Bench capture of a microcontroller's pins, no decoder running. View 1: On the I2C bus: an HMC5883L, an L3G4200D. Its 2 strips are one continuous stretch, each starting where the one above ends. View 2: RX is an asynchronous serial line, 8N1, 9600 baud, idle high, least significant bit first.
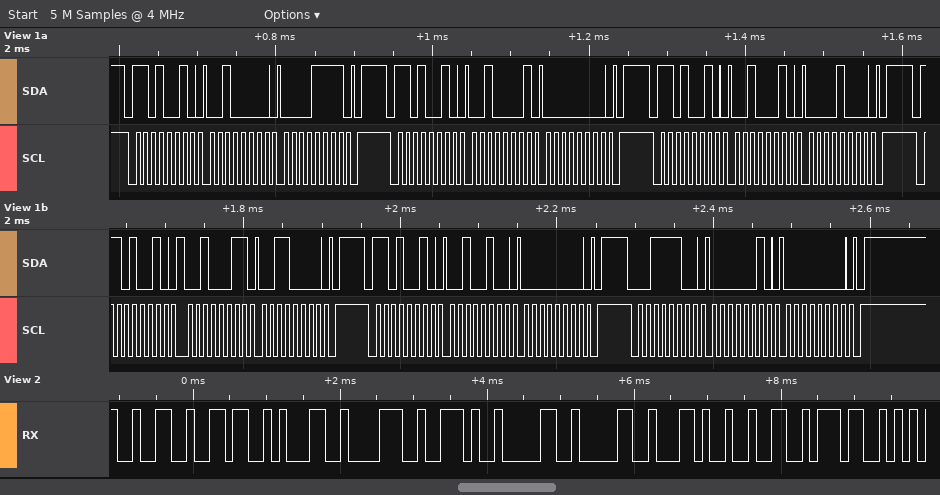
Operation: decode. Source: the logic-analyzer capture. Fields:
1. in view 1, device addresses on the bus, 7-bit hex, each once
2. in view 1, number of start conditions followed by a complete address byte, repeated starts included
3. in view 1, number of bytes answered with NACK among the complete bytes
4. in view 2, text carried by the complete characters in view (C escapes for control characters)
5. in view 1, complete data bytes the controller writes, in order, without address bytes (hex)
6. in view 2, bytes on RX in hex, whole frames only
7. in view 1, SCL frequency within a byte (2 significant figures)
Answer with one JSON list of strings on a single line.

["0x69 0x1E", "6", "0", "\"2618.00,27\"", "20 0F 21 00 22 08 23 30 24 00 02 00", "32 36 31 38 2E 30 30 2C 32 37", "100 kHz"]
